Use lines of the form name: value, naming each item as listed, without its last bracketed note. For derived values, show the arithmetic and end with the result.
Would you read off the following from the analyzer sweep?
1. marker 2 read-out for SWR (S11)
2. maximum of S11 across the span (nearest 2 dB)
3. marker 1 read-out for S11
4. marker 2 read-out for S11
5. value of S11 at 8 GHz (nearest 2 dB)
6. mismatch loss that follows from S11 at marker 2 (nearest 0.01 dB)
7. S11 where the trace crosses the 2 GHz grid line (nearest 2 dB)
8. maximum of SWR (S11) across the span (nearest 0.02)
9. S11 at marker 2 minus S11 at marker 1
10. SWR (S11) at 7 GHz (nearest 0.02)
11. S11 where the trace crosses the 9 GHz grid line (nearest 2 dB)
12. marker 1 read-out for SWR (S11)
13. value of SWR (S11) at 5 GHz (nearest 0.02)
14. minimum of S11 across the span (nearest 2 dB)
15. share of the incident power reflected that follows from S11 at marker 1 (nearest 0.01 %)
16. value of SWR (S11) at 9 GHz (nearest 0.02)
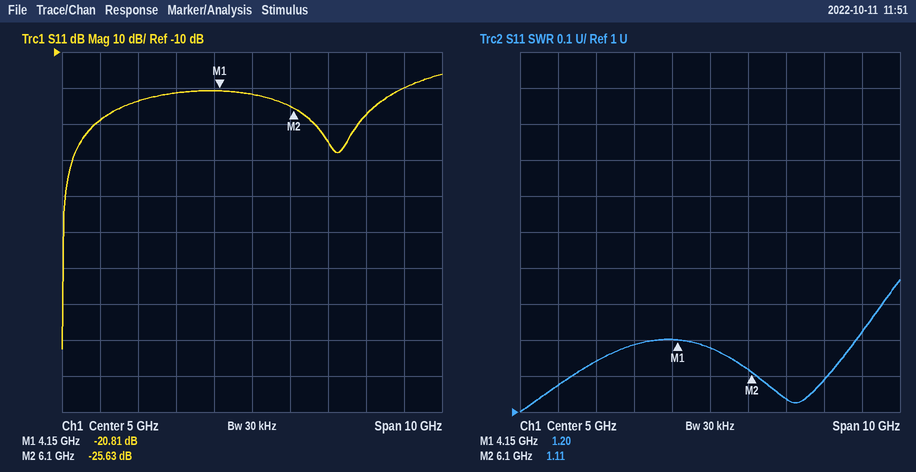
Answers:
marker 2 read-out for SWR: 1.11
maximum of S11 across the span: -16 dB
marker 1 read-out for S11: -20.81 dB
marker 2 read-out for S11: -25.63 dB
value of S11 at 8 GHz: -28 dB
mismatch loss that follows from S11 at marker 2: −10 log10(1 − 10^(-25.63/10)) ≈ 0.01 dB
S11 where the trace crosses the 2 GHz grid line: -24 dB
maximum of SWR (S11) across the span: 1.36
S11 at marker 2 minus S11 at marker 1: -25.63 − (-20.81) = -4.82 dB
SWR (S11) at 7 GHz: 1.04
S11 where the trace crosses the 9 GHz grid line: -20 dB
marker 1 read-out for SWR: 1.20
value of SWR (S11) at 5 GHz: 1.18
minimum of S11 across the span: -92 dB
share of the incident power reflected that follows from S11 at marker 1: 10^(-20.81/10) ≈ 0.83 %
value of SWR (S11) at 9 GHz: 1.22
